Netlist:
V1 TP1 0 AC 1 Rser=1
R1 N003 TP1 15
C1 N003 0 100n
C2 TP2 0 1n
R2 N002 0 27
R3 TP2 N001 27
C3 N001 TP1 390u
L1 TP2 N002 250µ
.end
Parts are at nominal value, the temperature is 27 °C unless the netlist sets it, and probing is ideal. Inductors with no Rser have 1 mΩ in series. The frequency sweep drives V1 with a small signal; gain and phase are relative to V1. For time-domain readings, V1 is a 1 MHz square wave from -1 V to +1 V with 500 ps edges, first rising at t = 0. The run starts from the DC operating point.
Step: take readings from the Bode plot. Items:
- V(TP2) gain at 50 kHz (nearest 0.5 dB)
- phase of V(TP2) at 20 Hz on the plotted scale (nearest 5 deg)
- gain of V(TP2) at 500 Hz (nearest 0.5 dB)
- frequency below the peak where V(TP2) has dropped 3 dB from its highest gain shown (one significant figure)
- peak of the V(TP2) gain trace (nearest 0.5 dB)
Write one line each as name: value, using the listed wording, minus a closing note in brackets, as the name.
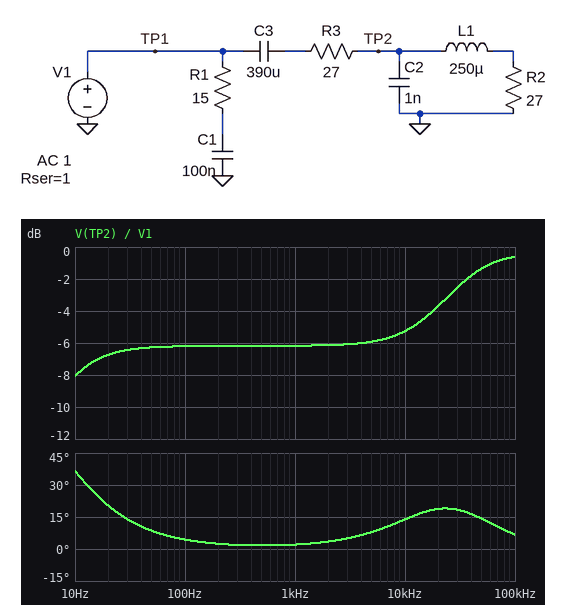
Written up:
V(TP2) gain at 50 kHz: -1.5 dB
phase of V(TP2) at 20 Hz on the plotted scale: 20 deg
gain of V(TP2) at 500 Hz: -6.0 dB
frequency below the peak where V(TP2) has dropped 3 dB from its highest gain shown: 20 kHz
peak of the V(TP2) gain trace: -0.5 dB
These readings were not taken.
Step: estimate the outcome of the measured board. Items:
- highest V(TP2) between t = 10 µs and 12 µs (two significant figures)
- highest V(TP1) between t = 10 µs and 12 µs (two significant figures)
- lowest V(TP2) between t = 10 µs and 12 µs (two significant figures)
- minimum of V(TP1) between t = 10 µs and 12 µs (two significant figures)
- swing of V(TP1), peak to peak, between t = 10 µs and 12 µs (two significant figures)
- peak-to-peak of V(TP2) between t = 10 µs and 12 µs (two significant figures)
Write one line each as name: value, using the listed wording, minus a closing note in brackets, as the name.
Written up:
highest V(TP2) between t = 10 µs and 12 µs: 1.5 V
highest V(TP1) between t = 10 µs and 12 µs: 930 mV
lowest V(TP2) between t = 10 µs and 12 µs: -420 mV
minimum of V(TP1) between t = 10 µs and 12 µs: -960 mV
swing of V(TP1), peak to peak, between t = 10 µs and 12 µs: 1.9 V
peak-to-peak of V(TP2) between t = 10 µs and 12 µs: 1.9 V
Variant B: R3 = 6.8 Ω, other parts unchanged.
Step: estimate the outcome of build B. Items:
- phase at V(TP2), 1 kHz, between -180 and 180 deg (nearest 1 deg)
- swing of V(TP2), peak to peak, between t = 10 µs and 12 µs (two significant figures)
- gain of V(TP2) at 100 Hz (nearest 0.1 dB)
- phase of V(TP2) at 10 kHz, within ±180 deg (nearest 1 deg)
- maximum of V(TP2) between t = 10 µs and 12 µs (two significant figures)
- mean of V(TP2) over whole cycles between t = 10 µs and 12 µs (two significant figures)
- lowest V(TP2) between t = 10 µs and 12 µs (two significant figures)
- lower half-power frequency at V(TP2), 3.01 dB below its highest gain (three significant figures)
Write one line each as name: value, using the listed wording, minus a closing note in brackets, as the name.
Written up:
phase at V(TP2), 1 kHz, between -180 and 180 deg: 1 deg
swing of V(TP2), peak to peak, between t = 10 µs and 12 µs: 1.9 V
gain of V(TP2) at 100 Hz: -2.3 dB
phase of V(TP2) at 10 kHz, within ±180 deg: 6 deg
maximum of V(TP2) between t = 10 µs and 12 µs: 1.8 V
mean of V(TP2) over whole cycles between t = 10 µs and 12 µs: 820 mV
lowest V(TP2) between t = 10 µs and 12 µs: -120 mV
lower half-power frequency at V(TP2), 3.01 dB below its highest gain: 21.4 Hz
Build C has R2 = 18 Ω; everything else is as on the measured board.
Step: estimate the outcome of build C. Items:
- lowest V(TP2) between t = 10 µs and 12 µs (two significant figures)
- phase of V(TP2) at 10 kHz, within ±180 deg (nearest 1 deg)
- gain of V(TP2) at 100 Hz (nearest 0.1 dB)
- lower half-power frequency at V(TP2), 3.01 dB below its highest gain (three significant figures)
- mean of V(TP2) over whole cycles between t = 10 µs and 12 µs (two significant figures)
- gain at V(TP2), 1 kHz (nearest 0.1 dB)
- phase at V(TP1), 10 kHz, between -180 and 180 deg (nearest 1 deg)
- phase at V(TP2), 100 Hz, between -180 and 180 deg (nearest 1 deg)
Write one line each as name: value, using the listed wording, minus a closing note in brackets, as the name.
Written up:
lowest V(TP2) between t = 10 µs and 12 µs: -480 mV
phase of V(TP2) at 10 kHz, within ±180 deg: 22 deg
gain of V(TP2) at 100 Hz: -8.2 dB
lower half-power frequency at V(TP2), 3.01 dB below its highest gain: 21.4 kHz
mean of V(TP2) over whole cycles between t = 10 µs and 12 µs: 480 mV
gain at V(TP2), 1 kHz: -8.1 dB
phase at V(TP1), 10 kHz, between -180 and 180 deg: 0 deg
phase at V(TP2), 100 Hz, between -180 and 180 deg: 5 deg
